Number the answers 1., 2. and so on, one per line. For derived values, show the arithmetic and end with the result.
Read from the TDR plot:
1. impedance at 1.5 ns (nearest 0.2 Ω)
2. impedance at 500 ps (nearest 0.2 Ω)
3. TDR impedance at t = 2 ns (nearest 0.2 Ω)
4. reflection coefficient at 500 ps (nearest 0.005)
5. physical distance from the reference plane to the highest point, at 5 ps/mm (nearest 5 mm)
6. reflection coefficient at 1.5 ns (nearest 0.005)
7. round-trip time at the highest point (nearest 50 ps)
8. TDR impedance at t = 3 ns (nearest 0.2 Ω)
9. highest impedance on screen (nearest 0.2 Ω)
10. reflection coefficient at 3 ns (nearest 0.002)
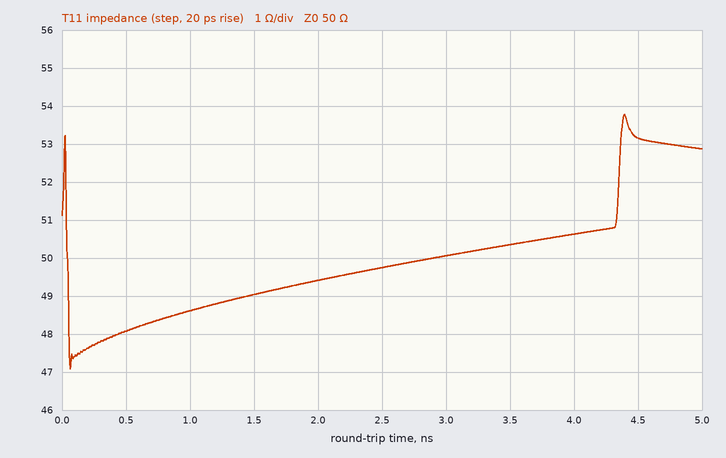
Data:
1. 49.0 Ω
2. 48.0 Ω
3. 49.4 Ω
4. (48 − 50)/(48 + 50) ≈ -0.020
5. 4.40 ns / 2 / 5 ps/mm ≈ 440 mm
6. (49 − 50)/(49 + 50) ≈ -0.010
7. 4.40 ns
8. 50.0 Ω
9. 53.8 Ω
10. (50 − 50)/(50 + 50) ≈ 0.000
